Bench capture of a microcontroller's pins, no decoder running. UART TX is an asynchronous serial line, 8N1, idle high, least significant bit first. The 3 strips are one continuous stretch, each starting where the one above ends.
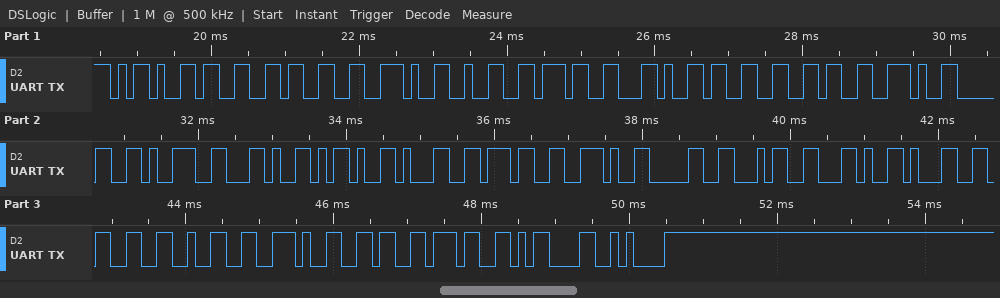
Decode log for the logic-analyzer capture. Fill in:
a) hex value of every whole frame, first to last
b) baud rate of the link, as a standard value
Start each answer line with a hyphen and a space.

- 0x2D 0x33 0x33 0x2E 0x32 0x37 0x2C 0x33 0x36 0x2E 0x30 0x39 0x2C 0x2D 0x31 0x37 0x2E 0x30 0x34 0x2C 0x31 0x33 0x32 0x2E 0x36 0x37 0x0D 0x0A
- 9600 baud
